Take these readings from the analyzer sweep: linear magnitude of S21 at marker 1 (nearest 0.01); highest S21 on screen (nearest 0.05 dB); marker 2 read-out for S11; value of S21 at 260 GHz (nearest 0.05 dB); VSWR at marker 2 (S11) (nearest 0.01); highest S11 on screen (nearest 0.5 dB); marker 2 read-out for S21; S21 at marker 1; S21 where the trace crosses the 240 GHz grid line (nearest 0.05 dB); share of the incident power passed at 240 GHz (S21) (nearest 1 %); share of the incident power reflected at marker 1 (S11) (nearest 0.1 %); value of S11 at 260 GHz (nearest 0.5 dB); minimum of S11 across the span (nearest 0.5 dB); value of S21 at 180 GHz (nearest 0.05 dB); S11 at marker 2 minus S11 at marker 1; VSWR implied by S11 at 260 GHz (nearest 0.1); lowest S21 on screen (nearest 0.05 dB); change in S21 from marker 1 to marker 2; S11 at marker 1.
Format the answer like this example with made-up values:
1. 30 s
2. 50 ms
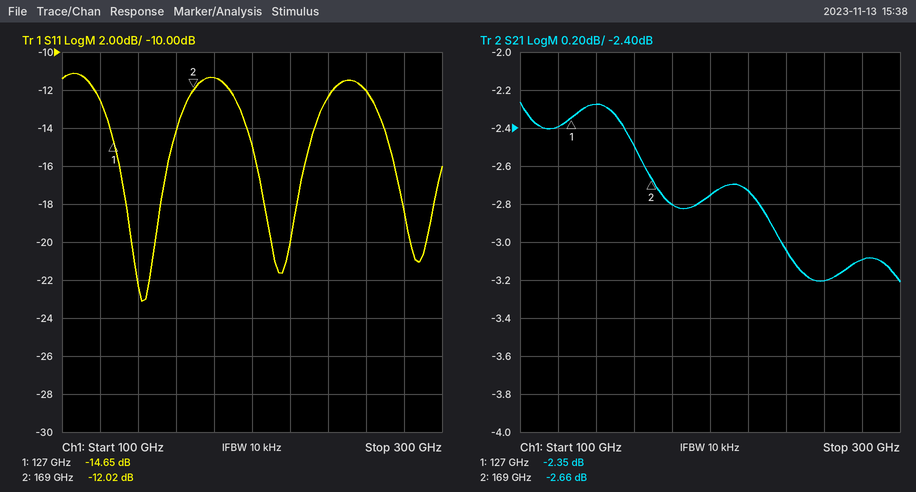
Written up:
1. 0.76
2. -2.25 dB
3. -12.02 dB
4. -3.20 dB
5. 1.67
6. -11.0 dB
7. -2.66 dB
8. -2.35 dB
9. -3.05 dB
10. 50 %
11. 3.4 %
12. -12.0 dB
13. -23.0 dB
14. -2.80 dB
15. 2.63 dB
16. 1.7
17. -3.20 dB
18. -0.31 dB
19. -14.65 dB
